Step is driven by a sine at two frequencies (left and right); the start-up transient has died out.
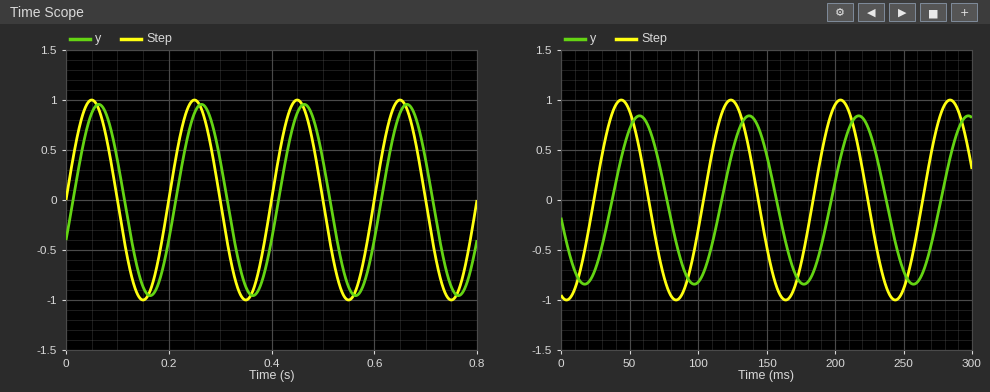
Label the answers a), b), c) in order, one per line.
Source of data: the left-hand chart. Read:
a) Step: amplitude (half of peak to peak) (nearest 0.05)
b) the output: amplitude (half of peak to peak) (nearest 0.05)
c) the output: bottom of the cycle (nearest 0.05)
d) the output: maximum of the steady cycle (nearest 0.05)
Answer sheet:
a) 1.00
b) 0.95
c) -0.95
d) 0.95
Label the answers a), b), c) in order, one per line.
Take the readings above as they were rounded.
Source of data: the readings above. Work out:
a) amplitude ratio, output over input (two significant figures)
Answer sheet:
a) 0.95
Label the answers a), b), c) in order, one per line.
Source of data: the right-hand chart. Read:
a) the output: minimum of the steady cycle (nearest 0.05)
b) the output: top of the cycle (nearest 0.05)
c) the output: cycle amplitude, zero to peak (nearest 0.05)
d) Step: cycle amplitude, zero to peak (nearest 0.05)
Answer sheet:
a) -0.85
b) 0.85
c) 0.85
d) 1.00
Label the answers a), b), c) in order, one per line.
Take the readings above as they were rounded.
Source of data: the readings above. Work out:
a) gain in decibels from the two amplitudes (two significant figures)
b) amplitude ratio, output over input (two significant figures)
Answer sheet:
a) -1.4 dB
b) 0.85
